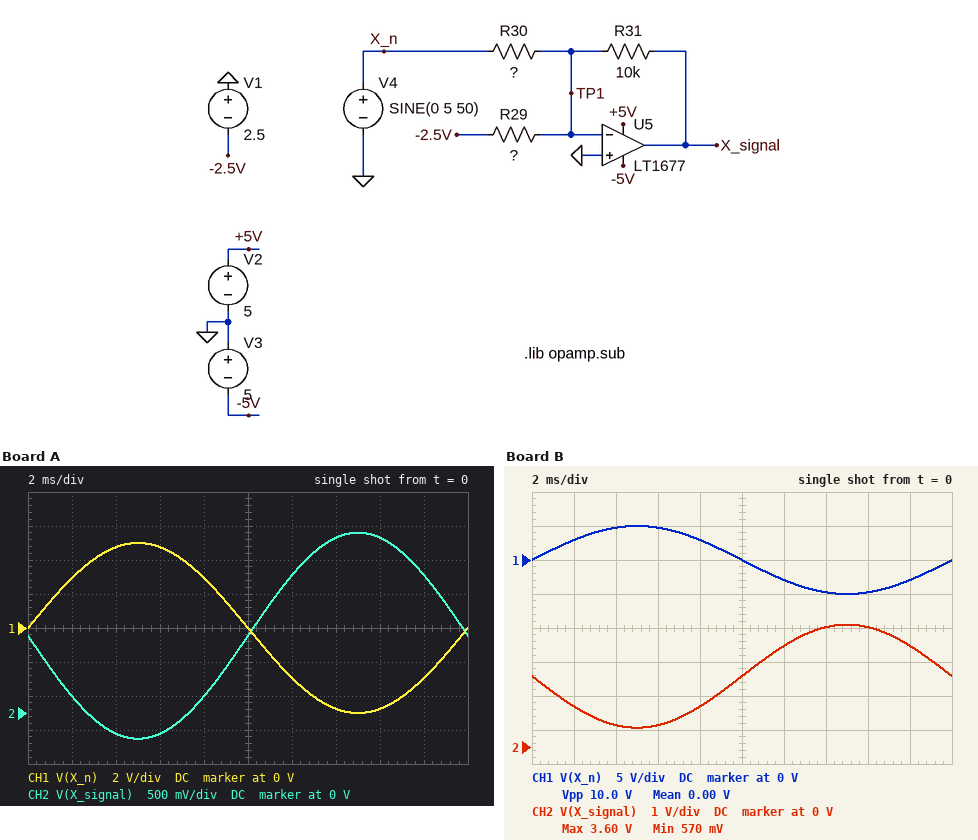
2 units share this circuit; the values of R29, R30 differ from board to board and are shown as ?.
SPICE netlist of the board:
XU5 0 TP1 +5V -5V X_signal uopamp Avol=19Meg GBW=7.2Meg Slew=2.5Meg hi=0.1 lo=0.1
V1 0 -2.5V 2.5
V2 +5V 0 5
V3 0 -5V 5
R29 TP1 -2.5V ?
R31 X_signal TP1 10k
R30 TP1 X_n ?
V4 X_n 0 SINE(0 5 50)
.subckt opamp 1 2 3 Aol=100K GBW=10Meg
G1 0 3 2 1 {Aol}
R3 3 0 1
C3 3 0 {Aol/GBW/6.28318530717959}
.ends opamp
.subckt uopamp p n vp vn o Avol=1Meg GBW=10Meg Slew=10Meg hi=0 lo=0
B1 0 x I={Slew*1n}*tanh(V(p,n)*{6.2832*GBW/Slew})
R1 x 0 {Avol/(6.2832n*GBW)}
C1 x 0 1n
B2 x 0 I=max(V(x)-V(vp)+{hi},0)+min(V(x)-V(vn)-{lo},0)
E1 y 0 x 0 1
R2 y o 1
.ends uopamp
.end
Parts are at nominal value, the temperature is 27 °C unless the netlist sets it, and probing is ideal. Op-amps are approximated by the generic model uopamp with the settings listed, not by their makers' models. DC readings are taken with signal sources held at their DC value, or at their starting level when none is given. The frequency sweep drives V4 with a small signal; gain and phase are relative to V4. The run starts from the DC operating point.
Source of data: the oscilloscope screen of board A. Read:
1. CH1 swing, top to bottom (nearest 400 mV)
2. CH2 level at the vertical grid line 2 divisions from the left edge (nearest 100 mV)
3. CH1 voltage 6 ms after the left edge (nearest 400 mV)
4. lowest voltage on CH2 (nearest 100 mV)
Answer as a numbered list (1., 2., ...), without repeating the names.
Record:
1. 10.0 V
2. -300 mV
3. 4.8 V
4. -400 mV
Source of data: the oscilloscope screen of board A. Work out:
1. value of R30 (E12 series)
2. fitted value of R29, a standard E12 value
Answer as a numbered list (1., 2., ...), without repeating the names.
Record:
1. 33 kΩ
2. 22 kΩ
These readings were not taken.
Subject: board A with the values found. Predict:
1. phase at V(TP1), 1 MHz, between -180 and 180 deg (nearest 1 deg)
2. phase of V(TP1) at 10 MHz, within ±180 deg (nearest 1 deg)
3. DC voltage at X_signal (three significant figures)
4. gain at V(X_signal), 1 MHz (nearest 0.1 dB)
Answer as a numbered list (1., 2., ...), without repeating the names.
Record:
1. 76 deg
2. 22 deg
3. 1.14 V
4. -10.6 dB
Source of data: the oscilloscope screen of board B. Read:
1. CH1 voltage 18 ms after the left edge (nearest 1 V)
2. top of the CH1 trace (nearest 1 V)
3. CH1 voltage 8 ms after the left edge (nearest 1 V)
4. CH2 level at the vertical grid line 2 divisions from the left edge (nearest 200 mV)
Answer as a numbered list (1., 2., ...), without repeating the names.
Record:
1. -3 V
2. 5 V
3. 3 V
4. 600 mV
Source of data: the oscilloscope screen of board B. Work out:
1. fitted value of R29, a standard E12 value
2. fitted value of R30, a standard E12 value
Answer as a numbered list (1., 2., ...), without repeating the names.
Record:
1. 12 kΩ
2. 33 kΩ
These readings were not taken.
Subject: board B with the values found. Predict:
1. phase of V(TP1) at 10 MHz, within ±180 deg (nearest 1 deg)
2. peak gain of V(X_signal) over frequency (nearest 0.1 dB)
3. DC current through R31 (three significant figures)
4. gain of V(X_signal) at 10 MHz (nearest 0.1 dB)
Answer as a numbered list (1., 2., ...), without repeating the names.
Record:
1. 19 deg
2. -10.4 dB
3. 208 µA
4. -20.3 dB
